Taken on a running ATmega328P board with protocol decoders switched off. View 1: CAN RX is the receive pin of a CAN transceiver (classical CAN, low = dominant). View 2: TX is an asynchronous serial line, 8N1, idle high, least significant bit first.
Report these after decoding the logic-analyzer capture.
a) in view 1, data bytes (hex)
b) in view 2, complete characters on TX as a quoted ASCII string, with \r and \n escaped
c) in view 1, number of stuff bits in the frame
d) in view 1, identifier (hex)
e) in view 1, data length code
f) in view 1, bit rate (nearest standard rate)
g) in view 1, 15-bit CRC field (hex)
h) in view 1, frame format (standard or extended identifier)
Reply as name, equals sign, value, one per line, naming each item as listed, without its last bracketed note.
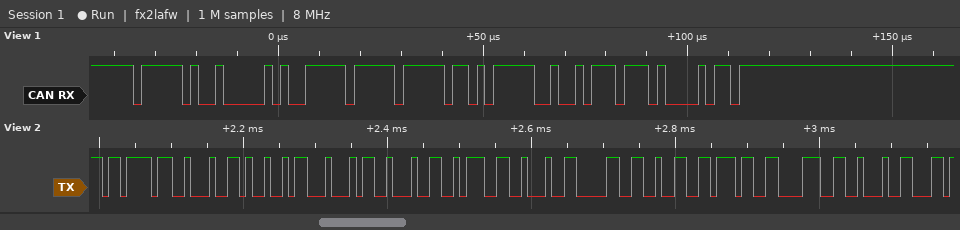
in view 1, data bytes = FF FF AF A5
in view 2, complete characters on TX as a quoted ASCII string, with \r and \n escaped = "{\"ID\":\"0278\""
in view 1, number of stuff bits in the frame = 6
in view 1, identifier = 0x7E4
in view 1, data length code = 4
in view 1, bit rate = 500 kbit/s
in view 1, 15-bit CRC field = 0x6E85
in view 1, frame format = standard
